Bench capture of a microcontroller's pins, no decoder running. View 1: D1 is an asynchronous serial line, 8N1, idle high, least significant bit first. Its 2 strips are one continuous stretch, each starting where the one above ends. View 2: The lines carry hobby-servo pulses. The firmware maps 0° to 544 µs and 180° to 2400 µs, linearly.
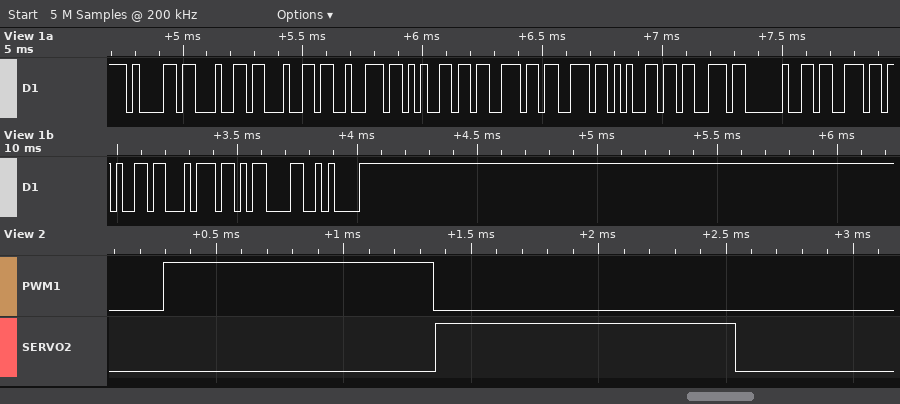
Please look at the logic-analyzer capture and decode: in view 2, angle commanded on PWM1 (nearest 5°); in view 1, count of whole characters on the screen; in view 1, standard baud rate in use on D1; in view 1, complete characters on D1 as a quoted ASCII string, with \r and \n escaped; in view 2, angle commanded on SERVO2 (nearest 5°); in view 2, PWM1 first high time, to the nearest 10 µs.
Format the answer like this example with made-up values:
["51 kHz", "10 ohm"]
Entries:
["50°", "15", "38400 baud", "\"addresses set\\r\\n\"", "60°", "1060 µs"]
